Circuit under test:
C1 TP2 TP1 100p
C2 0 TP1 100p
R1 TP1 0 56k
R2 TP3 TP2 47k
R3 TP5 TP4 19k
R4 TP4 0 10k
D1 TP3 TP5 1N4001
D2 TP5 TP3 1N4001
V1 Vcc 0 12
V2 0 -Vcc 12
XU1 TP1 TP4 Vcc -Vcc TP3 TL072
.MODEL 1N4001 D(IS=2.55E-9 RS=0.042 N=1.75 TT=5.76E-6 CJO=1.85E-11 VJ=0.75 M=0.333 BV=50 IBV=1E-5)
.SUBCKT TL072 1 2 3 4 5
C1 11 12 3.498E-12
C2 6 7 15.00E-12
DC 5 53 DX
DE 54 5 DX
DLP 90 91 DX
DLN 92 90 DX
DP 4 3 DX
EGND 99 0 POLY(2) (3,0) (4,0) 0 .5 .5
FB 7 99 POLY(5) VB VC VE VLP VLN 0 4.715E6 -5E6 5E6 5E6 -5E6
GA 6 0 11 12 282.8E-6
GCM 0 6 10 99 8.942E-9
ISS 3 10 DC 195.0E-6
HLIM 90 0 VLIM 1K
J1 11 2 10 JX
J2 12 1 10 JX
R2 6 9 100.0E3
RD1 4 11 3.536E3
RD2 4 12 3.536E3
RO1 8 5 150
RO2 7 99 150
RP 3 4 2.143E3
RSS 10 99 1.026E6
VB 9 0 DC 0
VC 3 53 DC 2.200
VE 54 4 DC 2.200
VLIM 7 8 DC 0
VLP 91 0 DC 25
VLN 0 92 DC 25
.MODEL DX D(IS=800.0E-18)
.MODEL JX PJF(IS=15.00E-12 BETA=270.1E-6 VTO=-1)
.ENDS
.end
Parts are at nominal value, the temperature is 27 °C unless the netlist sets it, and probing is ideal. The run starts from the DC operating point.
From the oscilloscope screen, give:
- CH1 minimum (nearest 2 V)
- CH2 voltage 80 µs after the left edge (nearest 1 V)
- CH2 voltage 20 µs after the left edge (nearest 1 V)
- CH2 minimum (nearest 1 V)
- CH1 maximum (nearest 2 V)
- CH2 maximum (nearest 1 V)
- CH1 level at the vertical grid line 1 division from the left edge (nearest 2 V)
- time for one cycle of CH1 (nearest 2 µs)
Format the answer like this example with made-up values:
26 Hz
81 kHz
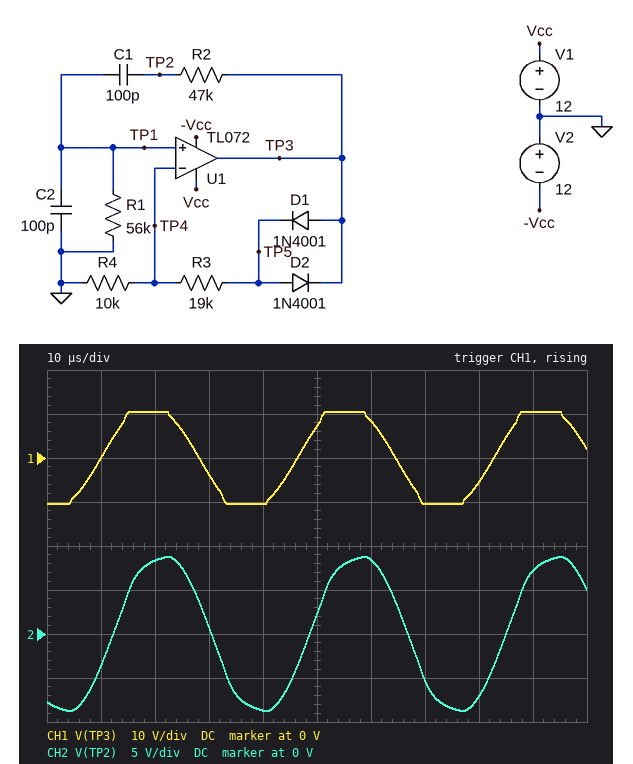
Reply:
-10 V
-7 V
8 V
-9 V
10 V
9 V
0 V
36 µs
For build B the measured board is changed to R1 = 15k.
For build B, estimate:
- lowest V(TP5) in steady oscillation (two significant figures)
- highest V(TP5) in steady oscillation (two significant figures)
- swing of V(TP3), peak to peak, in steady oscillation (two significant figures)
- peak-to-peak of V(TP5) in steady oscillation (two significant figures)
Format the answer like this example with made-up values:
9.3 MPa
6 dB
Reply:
-370 mV
370 mV
1.4 V
750 mV
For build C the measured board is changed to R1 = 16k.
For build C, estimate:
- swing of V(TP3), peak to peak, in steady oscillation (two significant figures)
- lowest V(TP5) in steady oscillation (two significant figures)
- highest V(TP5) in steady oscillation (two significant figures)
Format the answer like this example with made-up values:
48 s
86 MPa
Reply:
1.5 V
-420 mV
420 mV
